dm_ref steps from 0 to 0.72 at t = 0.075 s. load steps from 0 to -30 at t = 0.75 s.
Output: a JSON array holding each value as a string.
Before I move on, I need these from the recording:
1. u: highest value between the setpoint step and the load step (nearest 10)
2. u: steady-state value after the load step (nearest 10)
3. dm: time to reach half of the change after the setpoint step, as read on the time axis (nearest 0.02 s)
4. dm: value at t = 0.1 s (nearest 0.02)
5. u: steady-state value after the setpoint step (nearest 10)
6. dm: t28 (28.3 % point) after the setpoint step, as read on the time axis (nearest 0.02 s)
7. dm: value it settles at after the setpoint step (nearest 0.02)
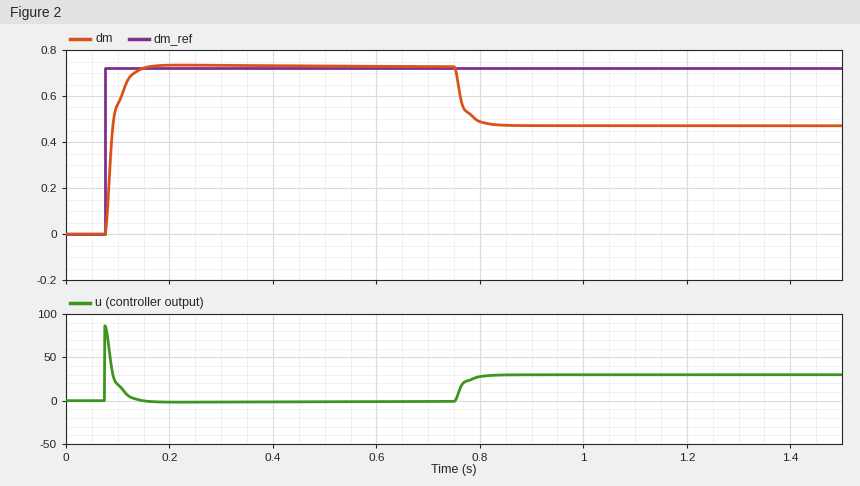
["90", "30", "0.08 s", "0.56", "0", "0.08 s", "0.72"]
